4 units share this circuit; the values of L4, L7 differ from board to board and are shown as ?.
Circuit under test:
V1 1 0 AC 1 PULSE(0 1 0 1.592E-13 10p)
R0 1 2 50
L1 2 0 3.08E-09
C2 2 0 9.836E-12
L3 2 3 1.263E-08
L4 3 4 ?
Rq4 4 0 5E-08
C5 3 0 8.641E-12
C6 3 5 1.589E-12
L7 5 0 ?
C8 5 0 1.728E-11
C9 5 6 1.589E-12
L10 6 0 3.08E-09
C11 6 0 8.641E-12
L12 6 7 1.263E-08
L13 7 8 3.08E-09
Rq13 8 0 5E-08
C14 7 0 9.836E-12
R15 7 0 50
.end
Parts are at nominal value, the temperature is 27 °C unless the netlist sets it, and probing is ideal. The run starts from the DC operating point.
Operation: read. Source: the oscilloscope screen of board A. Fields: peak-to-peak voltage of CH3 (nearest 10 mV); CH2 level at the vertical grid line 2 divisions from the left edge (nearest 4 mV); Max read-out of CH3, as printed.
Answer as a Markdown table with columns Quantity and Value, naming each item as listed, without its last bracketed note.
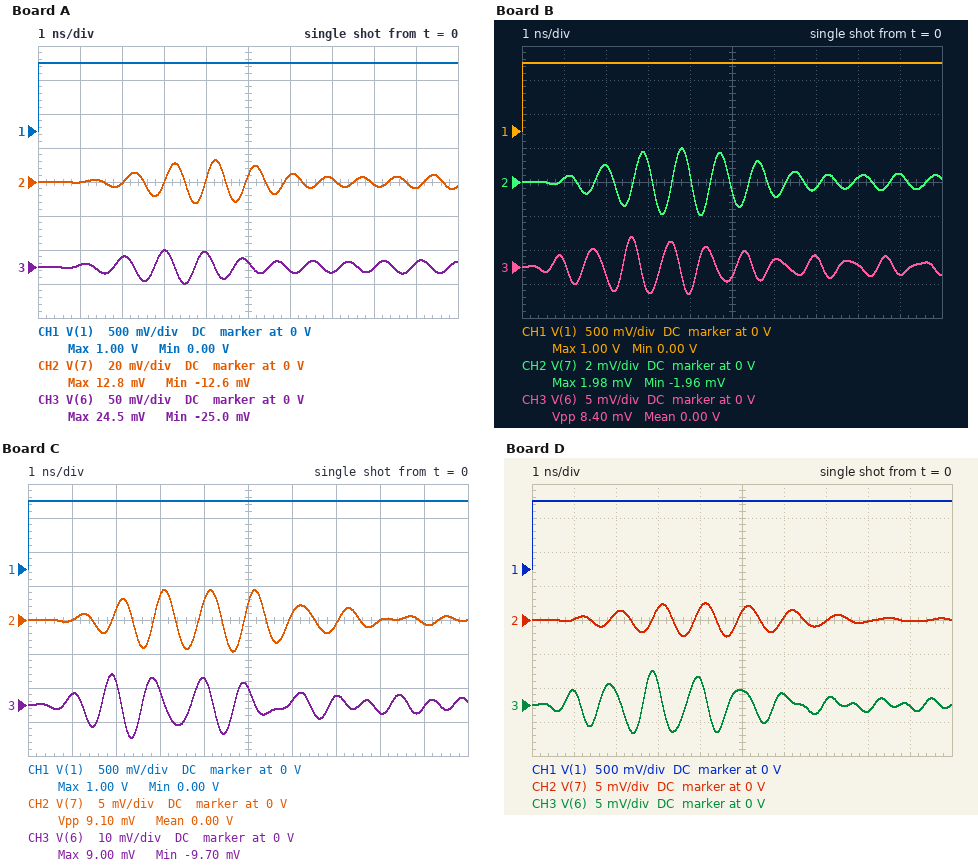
| Quantity | Value |
|---|---|
| peak-to-peak voltage of CH3 | 50 mV |
| CH2 level at the vertical grid line 2 divisions from the left edge | 0 V |
| Max read-out of CH3, as printed | 24.5 mV |
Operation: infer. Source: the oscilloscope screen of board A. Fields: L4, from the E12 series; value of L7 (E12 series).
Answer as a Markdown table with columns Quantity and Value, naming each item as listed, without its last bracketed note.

| Quantity | Value |
|---|---|
| L4, from the E12 series | 4.7 nH |
| value of L7 | 1 nH |
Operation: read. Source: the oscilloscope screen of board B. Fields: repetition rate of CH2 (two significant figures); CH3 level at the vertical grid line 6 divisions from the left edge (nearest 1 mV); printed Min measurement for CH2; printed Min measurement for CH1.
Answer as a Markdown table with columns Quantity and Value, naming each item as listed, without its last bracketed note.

| Quantity | Value |
|---|---|
| repetition rate of CH2 | 1.1 GHz |
| CH3 level at the vertical grid line 6 divisions from the left edge | 1 mV |
| printed Min measurement for CH2 | -1.96 mV |
| printed Min measurement for CH1 | 0.00 V |
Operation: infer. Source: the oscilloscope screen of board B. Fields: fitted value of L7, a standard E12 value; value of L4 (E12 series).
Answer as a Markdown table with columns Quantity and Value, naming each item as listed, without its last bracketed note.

| Quantity | Value |
|---|---|
| fitted value of L7, a standard E12 value | 390 pH |
| value of L4 | 2.2 nH |
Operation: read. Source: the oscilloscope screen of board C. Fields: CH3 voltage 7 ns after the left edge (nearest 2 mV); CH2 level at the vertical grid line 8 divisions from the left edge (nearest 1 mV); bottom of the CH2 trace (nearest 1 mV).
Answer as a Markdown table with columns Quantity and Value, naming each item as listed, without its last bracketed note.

| Quantity | Value |
|---|---|
| CH3 voltage 7 ns after the left edge | 2 mV |
| CH2 level at the vertical grid line 8 divisions from the left edge | 0 V |
| bottom of the CH2 trace | -5 mV |
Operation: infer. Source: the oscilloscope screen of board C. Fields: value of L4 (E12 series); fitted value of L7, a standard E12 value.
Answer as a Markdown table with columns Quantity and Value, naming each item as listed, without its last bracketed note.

| Quantity | Value |
|---|---|
| value of L4 | 3.9 nH |
| fitted value of L7, a standard E12 value | 680 pH |
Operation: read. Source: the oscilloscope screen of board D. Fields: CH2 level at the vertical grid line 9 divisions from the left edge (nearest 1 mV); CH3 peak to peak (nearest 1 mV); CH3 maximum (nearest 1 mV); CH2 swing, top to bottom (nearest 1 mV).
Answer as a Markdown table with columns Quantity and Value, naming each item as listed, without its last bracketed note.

| Quantity | Value |
|---|---|
| CH2 level at the vertical grid line 9 divisions from the left edge | 0 V |
| CH3 peak to peak | 9 mV |
| CH3 maximum | 5 mV |
| CH2 swing, top to bottom | 5 mV |
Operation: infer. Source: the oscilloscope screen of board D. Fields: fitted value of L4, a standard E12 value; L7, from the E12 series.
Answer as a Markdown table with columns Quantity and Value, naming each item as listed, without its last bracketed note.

| Quantity | Value |
|---|---|
| fitted value of L4, a standard E12 value | 3.9 nH |
| L7, from the E12 series | 470 pH |
